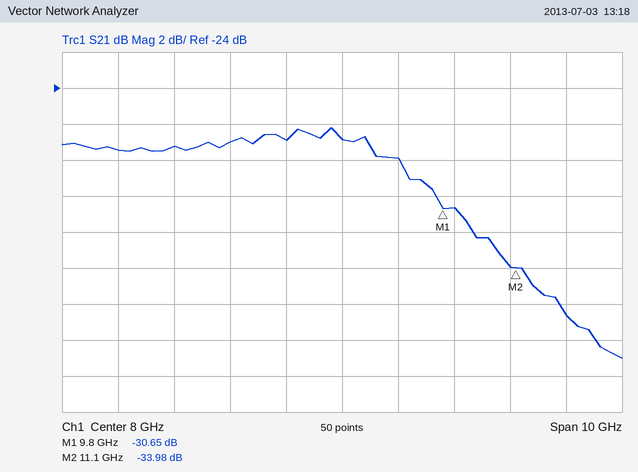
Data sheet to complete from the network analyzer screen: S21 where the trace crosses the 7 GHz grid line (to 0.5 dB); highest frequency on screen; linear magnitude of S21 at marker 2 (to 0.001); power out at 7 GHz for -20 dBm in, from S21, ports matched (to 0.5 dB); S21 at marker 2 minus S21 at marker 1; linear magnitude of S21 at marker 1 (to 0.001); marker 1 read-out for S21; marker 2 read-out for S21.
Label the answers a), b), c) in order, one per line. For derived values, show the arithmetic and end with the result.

a) -27.0 dB
b) 13 GHz
c) 10^(-33.98/20) ≈ 0.020
d) -20 dBm + (-27.0 dB) = -47.0 dBm
e) -33.98 − (-30.65) = -3.33 dB
f) 10^(-30.65/20) ≈ 0.029
g) -30.65 dB
h) -33.98 dB
